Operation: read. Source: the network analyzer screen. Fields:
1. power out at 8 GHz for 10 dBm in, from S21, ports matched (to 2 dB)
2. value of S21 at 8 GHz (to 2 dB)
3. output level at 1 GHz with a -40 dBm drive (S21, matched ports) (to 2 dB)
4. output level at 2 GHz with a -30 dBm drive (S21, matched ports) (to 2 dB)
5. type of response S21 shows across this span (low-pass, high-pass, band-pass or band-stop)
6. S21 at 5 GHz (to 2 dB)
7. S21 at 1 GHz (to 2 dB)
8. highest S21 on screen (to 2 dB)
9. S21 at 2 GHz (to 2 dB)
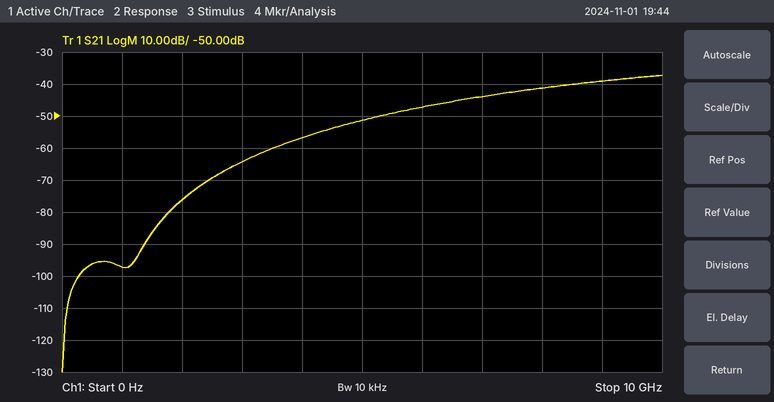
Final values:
-32 dBm
-42 dB
-138 dBm
-106 dBm
high-pass
-52 dB
-98 dB
-38 dB
-76 dB
